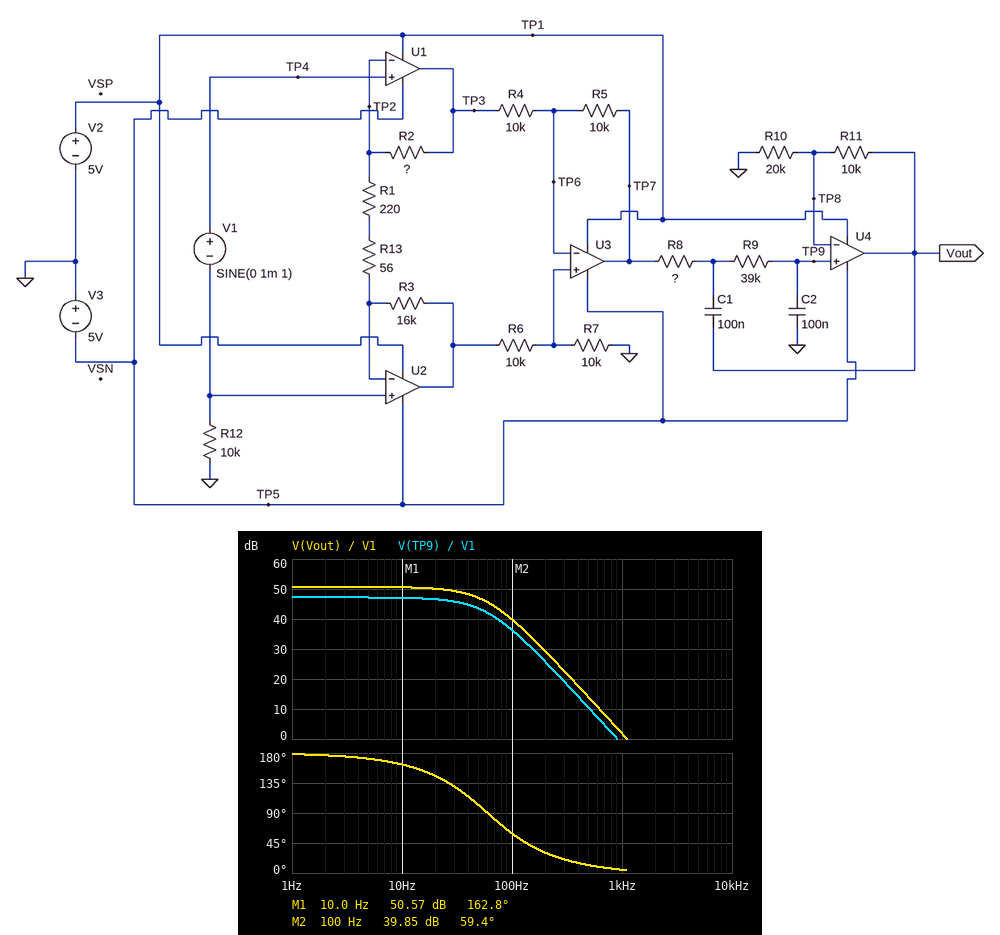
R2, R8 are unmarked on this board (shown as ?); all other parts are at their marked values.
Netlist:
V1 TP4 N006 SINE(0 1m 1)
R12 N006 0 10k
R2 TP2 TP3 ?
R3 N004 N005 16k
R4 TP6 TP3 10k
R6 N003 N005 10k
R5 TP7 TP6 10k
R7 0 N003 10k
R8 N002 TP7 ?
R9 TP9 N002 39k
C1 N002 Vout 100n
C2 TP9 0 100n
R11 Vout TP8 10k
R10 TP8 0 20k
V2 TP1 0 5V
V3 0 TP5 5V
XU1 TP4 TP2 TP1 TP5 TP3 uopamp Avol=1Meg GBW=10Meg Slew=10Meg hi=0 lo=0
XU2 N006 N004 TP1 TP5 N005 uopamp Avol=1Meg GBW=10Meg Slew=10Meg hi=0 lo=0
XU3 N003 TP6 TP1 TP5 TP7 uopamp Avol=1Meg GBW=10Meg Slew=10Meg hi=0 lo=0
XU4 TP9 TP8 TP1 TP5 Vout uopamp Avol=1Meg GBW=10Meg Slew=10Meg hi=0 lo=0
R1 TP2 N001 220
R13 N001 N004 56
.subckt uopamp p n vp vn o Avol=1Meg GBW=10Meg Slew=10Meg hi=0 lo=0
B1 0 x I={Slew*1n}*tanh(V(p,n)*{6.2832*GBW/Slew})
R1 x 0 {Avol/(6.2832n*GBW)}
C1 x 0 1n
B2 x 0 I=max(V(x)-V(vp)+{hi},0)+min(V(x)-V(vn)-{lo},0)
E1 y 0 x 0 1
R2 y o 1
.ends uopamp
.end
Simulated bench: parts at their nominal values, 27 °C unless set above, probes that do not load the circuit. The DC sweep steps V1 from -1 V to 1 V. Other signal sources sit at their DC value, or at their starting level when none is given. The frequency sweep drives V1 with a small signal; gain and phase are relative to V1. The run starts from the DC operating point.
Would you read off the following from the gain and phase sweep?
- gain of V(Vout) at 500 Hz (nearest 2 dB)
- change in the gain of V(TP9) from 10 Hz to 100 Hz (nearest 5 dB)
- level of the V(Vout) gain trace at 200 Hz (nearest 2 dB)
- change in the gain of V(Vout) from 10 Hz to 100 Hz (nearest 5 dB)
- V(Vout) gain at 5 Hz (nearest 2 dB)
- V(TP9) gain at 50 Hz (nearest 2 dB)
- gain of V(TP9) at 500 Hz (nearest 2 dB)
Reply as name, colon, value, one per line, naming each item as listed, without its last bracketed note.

gain of V(Vout) at 500 Hz: 14 dB
change in the gain of V(TP9) from 10 Hz to 100 Hz: -10 dB
level of the V(Vout) gain trace at 200 Hz: 30 dB
change in the gain of V(Vout) from 10 Hz to 100 Hz: -10 dB
V(Vout) gain at 5 Hz: 50 dB
V(TP9) gain at 50 Hz: 44 dB
gain of V(TP9) at 500 Hz: 10 dB
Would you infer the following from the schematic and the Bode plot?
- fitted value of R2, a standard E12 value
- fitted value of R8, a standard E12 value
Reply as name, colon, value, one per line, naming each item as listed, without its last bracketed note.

fitted value of R2, a standard E12 value: 47 kΩ
fitted value of R8, a standard E12 value: 18 kΩ
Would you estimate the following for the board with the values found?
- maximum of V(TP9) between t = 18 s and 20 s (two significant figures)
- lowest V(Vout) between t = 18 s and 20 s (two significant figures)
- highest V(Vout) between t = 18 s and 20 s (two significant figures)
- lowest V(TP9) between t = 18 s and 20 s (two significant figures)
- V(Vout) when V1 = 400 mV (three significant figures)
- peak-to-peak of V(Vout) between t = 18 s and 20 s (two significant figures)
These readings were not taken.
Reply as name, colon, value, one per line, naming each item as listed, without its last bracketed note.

maximum of V(TP9) between t = 18 s and 20 s: 230 mV
lowest V(Vout) between t = 18 s and 20 s: -340 mV
highest V(Vout) between t = 18 s and 20 s: 340 mV
lowest V(TP9) between t = 18 s and 20 s: -230 mV
V(Vout) when V1 = 400 mV: -5.01 V
peak-to-peak of V(Vout) between t = 18 s and 20 s: 690 mV
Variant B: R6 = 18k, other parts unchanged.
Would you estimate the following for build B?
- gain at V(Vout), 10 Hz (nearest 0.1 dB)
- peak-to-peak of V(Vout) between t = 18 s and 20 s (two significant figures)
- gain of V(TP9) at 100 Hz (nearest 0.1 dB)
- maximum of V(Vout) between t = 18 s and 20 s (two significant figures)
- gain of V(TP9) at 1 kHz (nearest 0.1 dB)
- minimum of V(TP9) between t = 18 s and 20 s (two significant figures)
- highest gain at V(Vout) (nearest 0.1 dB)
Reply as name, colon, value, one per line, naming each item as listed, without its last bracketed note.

gain at V(Vout), 10 Hz: 49.9 dB
peak-to-peak of V(Vout) between t = 18 s and 20 s: 640 mV
gain of V(TP9) at 100 Hz: 35.7 dB
maximum of V(Vout) between t = 18 s and 20 s: 320 mV
gain of V(TP9) at 1 kHz: -2.3 dB
minimum of V(TP9) between t = 18 s and 20 s: -210 mV
highest gain at V(Vout): 50.1 dB
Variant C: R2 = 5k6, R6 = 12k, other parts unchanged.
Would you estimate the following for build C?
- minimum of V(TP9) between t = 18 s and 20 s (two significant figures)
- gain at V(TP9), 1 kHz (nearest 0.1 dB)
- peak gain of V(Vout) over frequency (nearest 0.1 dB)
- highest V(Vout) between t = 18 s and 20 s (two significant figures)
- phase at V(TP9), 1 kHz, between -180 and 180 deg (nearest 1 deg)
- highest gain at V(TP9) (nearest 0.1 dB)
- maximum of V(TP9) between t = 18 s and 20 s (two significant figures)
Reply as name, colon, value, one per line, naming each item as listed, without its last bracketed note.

minimum of V(TP9) between t = 18 s and 20 s: -74 mV
gain at V(TP9), 1 kHz: -11.5 dB
peak gain of V(Vout) over frequency: 40.9 dB
highest V(Vout) between t = 18 s and 20 s: 110 mV
phase at V(TP9), 1 kHz, between -180 and 180 deg: 6 deg
highest gain at V(TP9): 37.4 dB
maximum of V(TP9) between t = 18 s and 20 s: 74 mV
